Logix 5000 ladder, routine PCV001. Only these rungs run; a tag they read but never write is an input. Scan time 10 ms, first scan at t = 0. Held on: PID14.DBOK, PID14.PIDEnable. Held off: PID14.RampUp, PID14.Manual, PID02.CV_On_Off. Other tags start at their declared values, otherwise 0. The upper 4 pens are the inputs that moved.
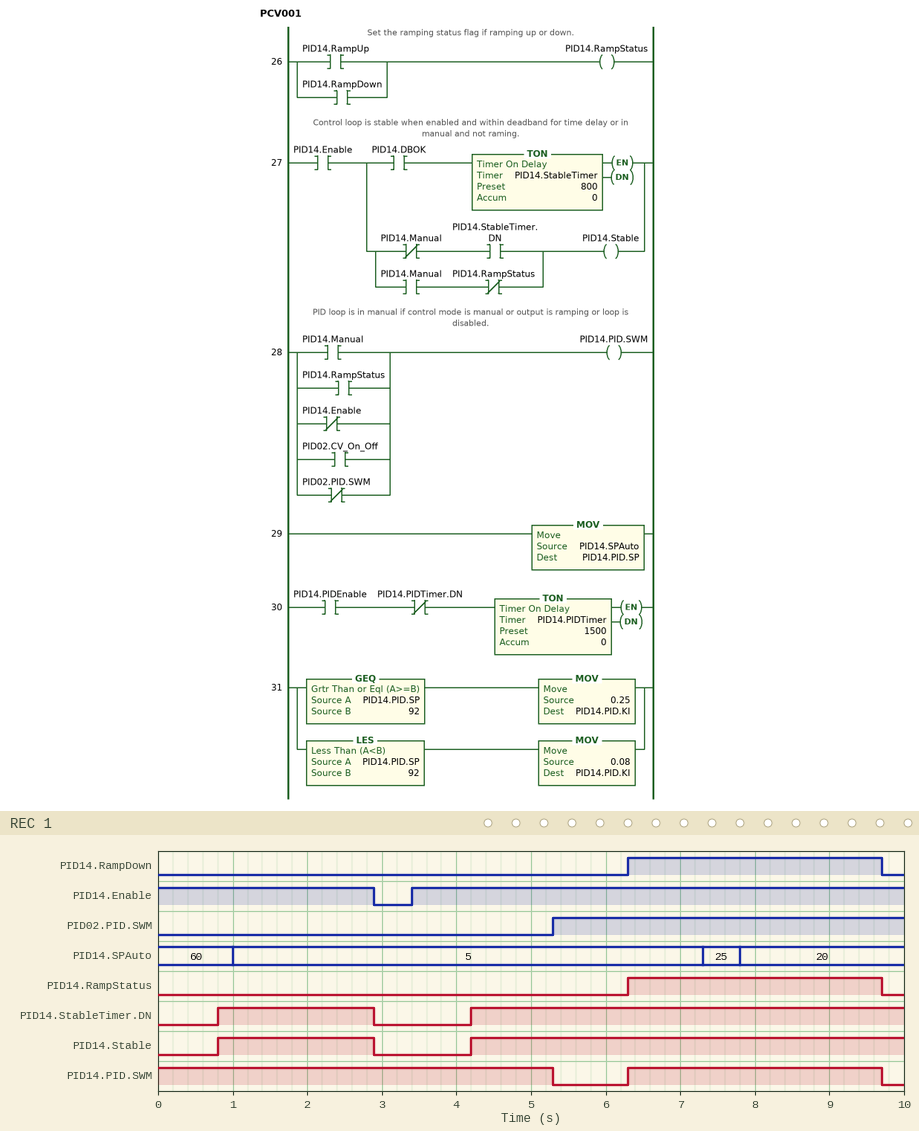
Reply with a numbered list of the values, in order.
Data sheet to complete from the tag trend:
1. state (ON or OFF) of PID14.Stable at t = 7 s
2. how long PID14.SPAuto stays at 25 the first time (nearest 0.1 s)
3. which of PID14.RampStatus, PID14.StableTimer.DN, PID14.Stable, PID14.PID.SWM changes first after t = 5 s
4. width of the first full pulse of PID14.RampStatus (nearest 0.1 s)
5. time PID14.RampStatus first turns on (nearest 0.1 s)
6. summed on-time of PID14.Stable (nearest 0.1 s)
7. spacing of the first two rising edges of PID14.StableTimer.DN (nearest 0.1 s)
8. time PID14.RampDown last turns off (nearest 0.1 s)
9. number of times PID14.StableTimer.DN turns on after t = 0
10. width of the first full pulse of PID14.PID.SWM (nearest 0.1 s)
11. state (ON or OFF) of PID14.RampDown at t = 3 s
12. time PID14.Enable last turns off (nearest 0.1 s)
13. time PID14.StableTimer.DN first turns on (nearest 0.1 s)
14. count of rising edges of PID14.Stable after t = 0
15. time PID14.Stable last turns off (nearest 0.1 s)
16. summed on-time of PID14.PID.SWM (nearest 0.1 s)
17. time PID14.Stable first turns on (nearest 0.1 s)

1. ON
2. 0.5 s
3. PID14.PID.SWM
4. 3.4 s
5. 6.3 s
6. 7.9 s
7. 3.4 s
8. 9.7 s
9. 2
10. 3.4 s
11. OFF
12. 2.9 s
13. 0.8 s
14. 2
15. 2.9 s
16. 8.7 s
17. 0.8 s
